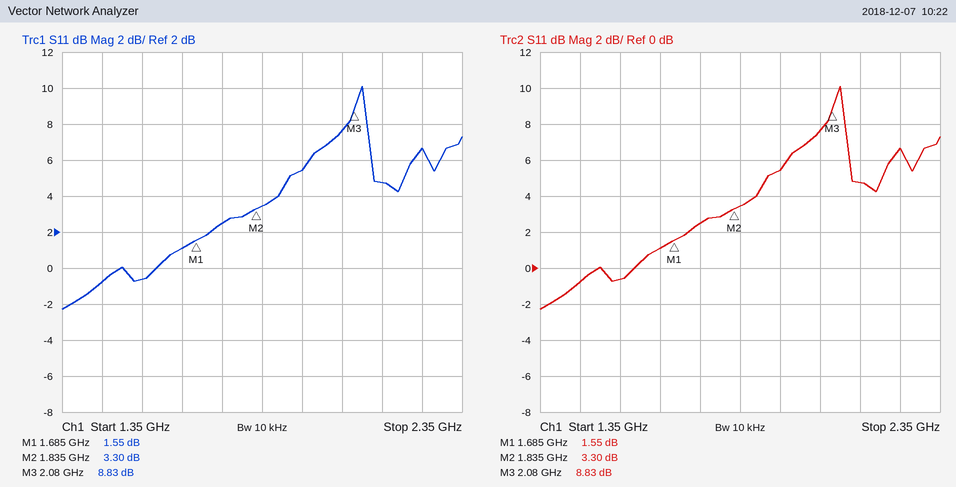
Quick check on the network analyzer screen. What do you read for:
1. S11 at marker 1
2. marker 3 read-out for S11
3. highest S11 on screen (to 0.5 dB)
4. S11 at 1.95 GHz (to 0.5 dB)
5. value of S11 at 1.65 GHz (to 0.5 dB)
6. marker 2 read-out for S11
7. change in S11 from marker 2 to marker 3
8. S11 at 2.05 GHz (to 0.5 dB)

1.55 dB
8.83 dB
10.0 dB
5.5 dB
1.0 dB
3.30 dB
5.53 dB
7.5 dB
